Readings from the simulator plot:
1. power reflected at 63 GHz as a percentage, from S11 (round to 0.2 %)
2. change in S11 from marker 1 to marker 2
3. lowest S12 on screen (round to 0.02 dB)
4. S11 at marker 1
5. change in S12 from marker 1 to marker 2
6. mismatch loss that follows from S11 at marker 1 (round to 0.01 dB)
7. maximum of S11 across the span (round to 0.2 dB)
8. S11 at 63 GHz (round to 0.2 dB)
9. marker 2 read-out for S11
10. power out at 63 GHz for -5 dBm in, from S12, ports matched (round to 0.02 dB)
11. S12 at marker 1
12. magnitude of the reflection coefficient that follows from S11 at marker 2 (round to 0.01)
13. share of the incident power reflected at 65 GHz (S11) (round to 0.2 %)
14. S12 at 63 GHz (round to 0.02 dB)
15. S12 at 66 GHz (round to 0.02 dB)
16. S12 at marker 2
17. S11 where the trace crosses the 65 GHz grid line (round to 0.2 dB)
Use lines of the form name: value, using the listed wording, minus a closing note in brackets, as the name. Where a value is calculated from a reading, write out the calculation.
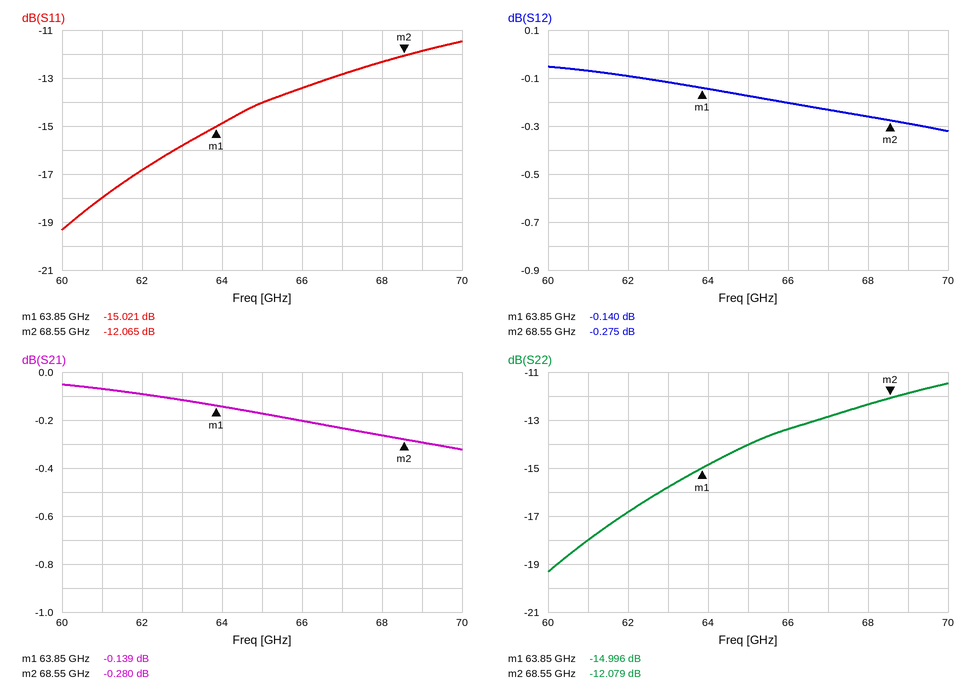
power reflected at 63 GHz as a percentage, from S11: 10^(-15.8/10) ≈ 2.6 %
change in S11 from marker 1 to marker 2: -12.065 − (-15.021) = 2.956 dB
lowest S12 on screen: -0.32 dB
S11 at marker 1: -15.021 dB
change in S12 from marker 1 to marker 2: -0.275 − (-0.14) = -0.135 dB
mismatch loss that follows from S11 at marker 1: −10 log10(1 − 10^(-15.021/10)) ≈ 0.14 dB
maximum of S11 across the span: -11.4 dB
S11 at 63 GHz: -15.8 dB
marker 2 read-out for S11: -12.065 dB
power out at 63 GHz for -5 dBm in, from S12, ports matched: -5 dBm + (-0.12 dB) = -5.12 dBm
S12 at marker 1: -0.140 dB
magnitude of the reflection coefficient that follows from S11 at marker 2: 10^(-12.065/20) ≈ 0.25
share of the incident power reflected at 65 GHz (S11): 10^(-14/10) ≈ 4.0 %
S12 at 63 GHz: -0.12 dB
S12 at 66 GHz: -0.20 dB
S12 at marker 2: -0.275 dB
S11 where the trace crosses the 65 GHz grid line: -14.0 dB
